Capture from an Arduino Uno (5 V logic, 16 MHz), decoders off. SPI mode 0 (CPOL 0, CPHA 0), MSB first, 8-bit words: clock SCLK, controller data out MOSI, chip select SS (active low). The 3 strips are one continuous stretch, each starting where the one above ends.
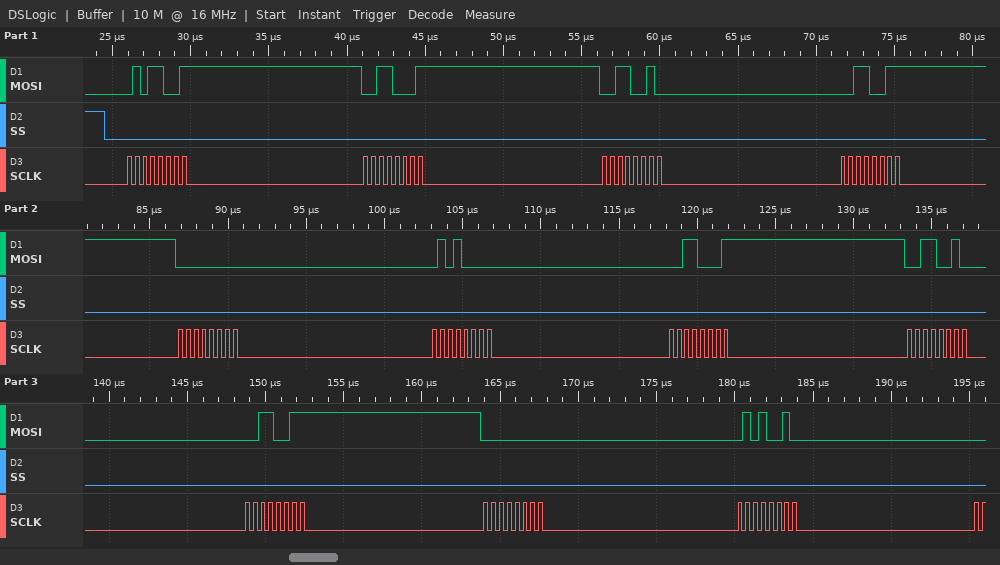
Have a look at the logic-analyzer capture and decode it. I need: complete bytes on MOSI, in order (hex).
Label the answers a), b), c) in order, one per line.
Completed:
a) 0x59 0x31 0x32 0x33 0x00 0x50 0x31 0x32 0x33 0x00 0x52
